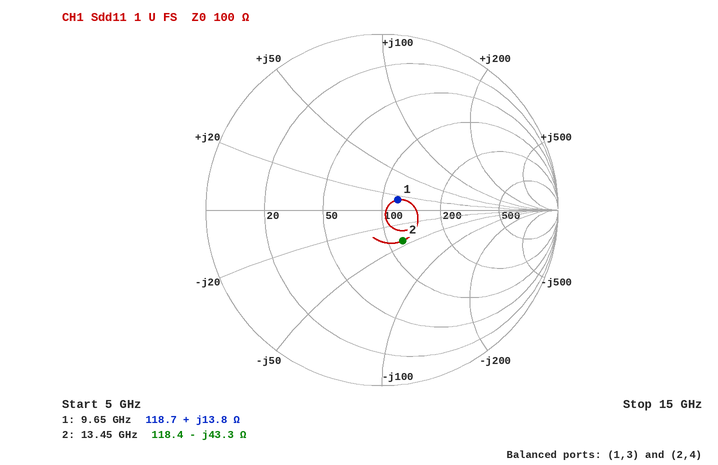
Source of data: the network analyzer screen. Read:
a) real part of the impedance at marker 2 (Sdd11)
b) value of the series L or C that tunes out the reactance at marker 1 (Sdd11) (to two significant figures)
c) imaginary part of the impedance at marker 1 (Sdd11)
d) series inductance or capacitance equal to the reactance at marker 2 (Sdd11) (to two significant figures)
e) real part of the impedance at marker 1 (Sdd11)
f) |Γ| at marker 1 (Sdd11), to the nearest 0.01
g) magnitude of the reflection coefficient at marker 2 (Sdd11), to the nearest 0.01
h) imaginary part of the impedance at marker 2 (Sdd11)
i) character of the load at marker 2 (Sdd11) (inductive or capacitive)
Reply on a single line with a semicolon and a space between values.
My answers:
118.4 Ω; 1.2 pF; +13.8 Ω; 270 fF; 118.7 Ω; 0.11; 0.21; -43.3 Ω; capacitive
